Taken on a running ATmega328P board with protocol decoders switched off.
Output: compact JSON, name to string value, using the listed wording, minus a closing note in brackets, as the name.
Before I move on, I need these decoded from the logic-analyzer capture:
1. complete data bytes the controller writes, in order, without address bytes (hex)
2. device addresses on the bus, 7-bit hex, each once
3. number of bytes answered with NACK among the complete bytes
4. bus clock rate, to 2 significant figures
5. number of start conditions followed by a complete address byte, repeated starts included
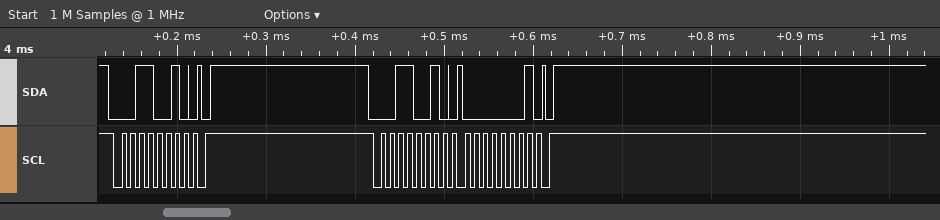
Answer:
{"complete data bytes the controller writes, in order, without address bytes": "01", "device addresses on the bus, 7-bit hex, each once": "0x19", "number of bytes answered with NACK among the complete bytes": "0", "bus clock rate, to 2 significant figures": "100 kHz", "number of start conditions followed by a complete address byte, repeated starts included": "2"}
